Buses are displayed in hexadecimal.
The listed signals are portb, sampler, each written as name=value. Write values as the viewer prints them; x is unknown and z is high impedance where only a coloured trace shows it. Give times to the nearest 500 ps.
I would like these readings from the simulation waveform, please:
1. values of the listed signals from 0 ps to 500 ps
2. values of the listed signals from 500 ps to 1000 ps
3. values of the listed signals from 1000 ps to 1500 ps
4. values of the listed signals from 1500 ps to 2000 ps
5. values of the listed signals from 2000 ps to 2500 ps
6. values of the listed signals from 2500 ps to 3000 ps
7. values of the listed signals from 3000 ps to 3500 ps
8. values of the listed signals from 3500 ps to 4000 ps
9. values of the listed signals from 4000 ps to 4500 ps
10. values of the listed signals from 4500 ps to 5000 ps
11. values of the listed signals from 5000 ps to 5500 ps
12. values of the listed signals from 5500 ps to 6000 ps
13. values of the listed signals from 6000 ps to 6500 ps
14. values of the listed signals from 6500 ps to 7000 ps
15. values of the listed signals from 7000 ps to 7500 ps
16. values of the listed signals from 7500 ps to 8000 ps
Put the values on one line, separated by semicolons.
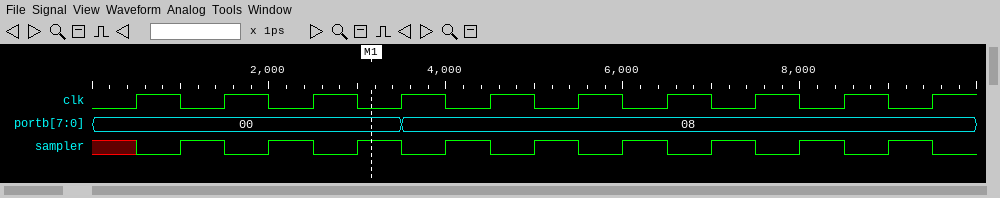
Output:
portb=00, sampler=x; portb=00, sampler=0; portb=00, sampler=1; portb=00, sampler=0; portb=00, sampler=1; portb=00, sampler=0; portb=00, sampler=1; portb=08, sampler=0; portb=08, sampler=1; portb=08, sampler=0; portb=08, sampler=1; portb=08, sampler=0; portb=08, sampler=1; portb=08, sampler=0; portb=08, sampler=1; portb=08, sampler=0
